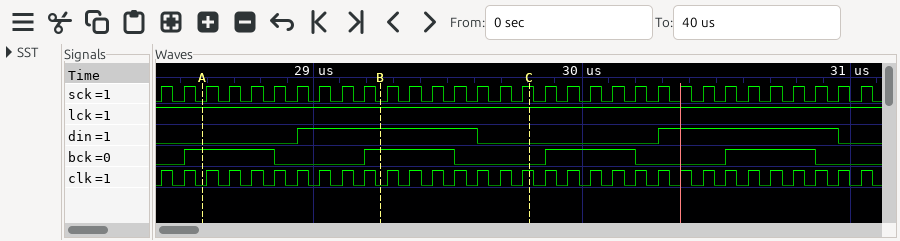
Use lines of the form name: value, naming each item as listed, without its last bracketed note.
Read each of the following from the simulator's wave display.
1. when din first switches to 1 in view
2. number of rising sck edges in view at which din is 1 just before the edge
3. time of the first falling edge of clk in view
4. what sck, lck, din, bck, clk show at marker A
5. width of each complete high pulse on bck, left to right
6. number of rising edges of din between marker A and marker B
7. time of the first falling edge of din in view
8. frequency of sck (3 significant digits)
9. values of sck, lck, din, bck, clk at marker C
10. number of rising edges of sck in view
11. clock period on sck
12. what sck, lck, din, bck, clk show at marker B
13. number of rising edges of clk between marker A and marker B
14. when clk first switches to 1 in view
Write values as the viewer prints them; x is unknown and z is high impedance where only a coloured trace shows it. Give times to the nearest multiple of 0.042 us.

when din first switches to 1 in view: 28.938 us
number of rising sck edges in view at which din is 1 just before the edge: 16
time of the first falling edge of clk in view: 28.476 us
what sck, lck, din, bck, clk show at marker A: sck=0, lck=1, din=0, bck=1, clk=0
width of each complete high pulse on bck, left to right: 0.336 us, 0.336 us, 0.336 us, 0.336 us
number of rising edges of din between marker A and marker B: 1
time of the first falling edge of din in view: 29.61 us
frequency of sck: 11.9 MHz
values of sck, lck, din, bck, clk at marker C: sck=1, lck=1, din=0, bck=0, clk=1
number of rising edges of sck in view: 32
clock period on sck: 0.084 us
what sck, lck, din, bck, clk show at marker B: sck=0, lck=1, din=1, bck=1, clk=0
number of rising edges of clk between marker A and marker B: 8
when clk first switches to 1 in view: 28.434 us
